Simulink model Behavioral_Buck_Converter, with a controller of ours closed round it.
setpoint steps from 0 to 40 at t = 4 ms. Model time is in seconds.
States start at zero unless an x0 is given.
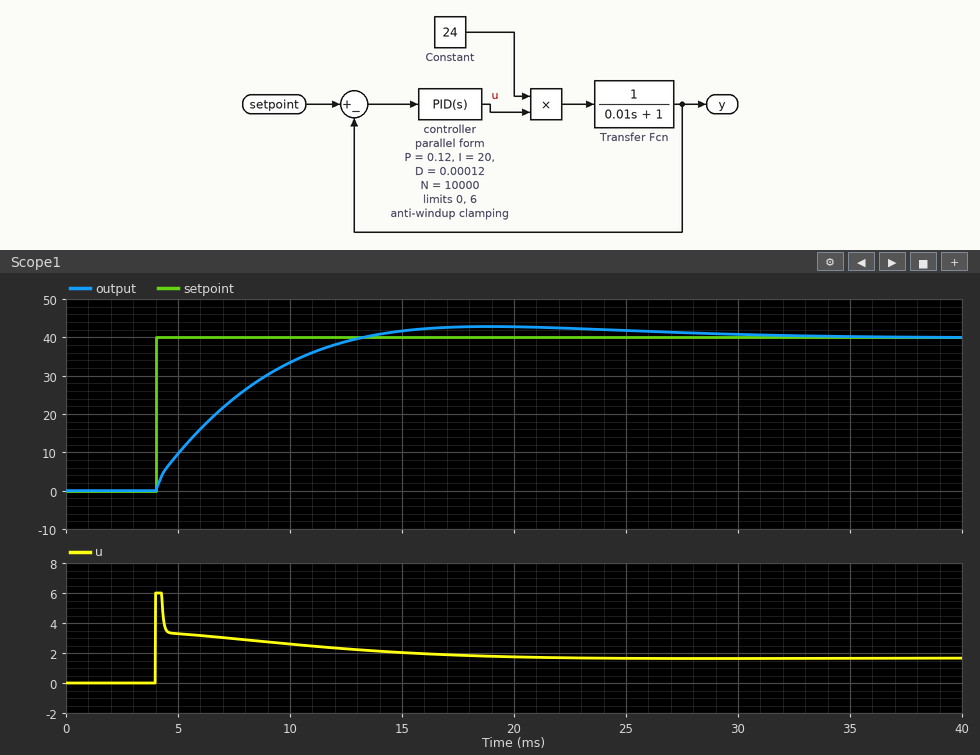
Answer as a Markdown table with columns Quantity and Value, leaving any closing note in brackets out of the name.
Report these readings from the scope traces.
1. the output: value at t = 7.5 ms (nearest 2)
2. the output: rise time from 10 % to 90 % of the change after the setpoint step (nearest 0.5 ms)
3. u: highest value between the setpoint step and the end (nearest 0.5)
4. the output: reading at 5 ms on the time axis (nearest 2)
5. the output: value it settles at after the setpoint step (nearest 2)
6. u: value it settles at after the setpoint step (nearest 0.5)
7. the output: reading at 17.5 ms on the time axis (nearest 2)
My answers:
| Quantity | Value |
|---|---|
| the output: value at t = 7.5 ms | 24 |
| the output: rise time from 10 % to 90 % of the change after the setpoint step | 6.5 ms |
| u: highest value between the setpoint step and the end | 6.0 |
| the output: reading at 5 ms on the time axis | 10 |
| the output: value it settles at after the setpoint step | 40 |
| u: value it settles at after the setpoint step | 1.5 |
| the output: reading at 17.5 ms on the time axis | 42 |
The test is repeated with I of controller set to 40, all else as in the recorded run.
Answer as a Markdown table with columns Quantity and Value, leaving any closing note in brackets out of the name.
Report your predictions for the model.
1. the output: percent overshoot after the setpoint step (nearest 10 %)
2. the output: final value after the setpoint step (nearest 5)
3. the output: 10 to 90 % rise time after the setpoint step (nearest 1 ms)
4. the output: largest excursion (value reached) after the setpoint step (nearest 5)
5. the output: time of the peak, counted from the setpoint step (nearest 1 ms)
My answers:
| Quantity | Value |
|---|---|
| the output: percent overshoot after the setpoint step | 20 % |
| the output: final value after the setpoint step | 40 |
| the output: 10 to 90 % rise time after the setpoint step | 5 ms |
| the output: largest excursion (value reached) after the setpoint step | 45 |
| the output: time of the peak, counted from the setpoint step | 10 ms |
